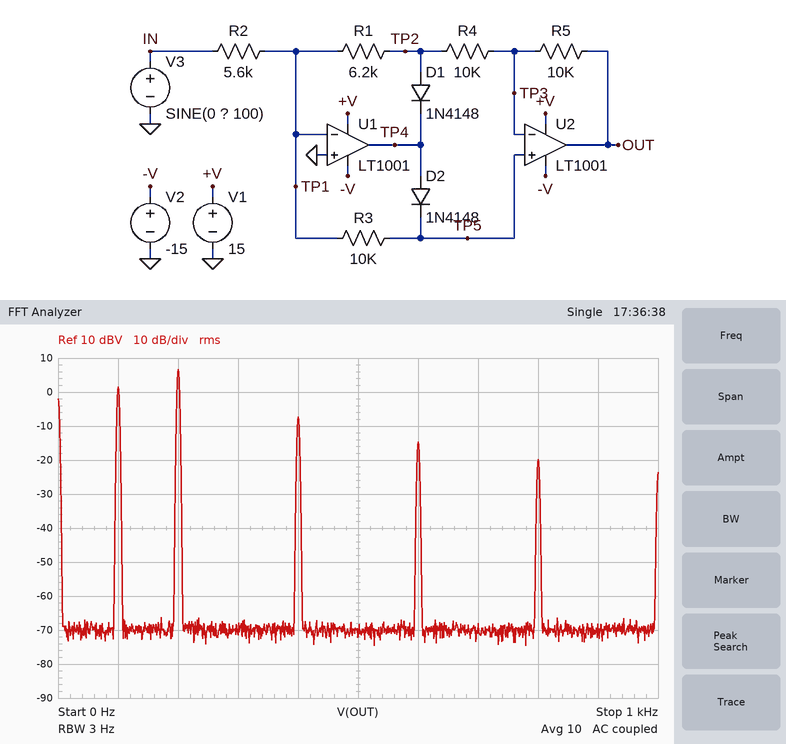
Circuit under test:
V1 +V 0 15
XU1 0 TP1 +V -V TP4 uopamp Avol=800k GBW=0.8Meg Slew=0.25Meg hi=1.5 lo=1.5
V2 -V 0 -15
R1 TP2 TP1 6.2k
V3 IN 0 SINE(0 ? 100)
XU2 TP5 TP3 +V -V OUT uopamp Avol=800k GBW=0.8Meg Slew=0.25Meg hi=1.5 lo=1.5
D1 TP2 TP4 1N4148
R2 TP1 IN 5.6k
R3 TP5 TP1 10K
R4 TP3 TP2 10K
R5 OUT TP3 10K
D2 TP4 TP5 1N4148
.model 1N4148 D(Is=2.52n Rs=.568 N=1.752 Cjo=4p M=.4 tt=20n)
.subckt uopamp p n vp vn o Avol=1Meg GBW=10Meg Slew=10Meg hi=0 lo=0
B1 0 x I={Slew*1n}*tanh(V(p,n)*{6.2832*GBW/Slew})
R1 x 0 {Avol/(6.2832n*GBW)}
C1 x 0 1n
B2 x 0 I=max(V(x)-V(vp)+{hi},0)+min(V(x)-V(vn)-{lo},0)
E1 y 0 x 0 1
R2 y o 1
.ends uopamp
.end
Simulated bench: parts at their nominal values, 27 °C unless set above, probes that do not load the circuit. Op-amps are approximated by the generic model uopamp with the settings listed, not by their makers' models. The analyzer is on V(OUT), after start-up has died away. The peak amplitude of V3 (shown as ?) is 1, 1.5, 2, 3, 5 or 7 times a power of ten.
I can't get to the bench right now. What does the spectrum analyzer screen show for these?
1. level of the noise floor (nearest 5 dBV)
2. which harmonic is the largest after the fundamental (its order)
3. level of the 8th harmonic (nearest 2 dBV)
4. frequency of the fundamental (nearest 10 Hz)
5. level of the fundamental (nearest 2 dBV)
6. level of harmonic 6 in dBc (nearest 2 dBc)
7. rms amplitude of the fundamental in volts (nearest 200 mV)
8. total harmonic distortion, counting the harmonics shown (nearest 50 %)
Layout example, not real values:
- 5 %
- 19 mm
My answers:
- -70 dBV
- 2
- -20 dBV
- 100 Hz
- 2 dBV
- -16 dBc
- 1.2 V
- 200 %
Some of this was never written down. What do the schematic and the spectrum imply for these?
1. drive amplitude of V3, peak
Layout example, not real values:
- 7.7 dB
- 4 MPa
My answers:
- 5 V
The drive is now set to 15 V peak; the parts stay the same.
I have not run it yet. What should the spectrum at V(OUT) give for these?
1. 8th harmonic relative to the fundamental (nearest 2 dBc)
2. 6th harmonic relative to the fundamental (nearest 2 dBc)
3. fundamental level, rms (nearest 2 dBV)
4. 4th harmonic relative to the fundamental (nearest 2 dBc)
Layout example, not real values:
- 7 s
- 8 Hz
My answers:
- -2 dBc
- 4 dBc
- -6 dBV
- 12 dBc
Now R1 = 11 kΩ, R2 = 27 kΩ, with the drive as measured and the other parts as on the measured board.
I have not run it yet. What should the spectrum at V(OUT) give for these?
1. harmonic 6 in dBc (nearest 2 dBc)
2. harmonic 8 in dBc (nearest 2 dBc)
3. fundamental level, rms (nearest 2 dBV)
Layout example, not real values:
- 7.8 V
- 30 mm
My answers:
- -2 dBc
- -8 dBc
- -24 dBV
